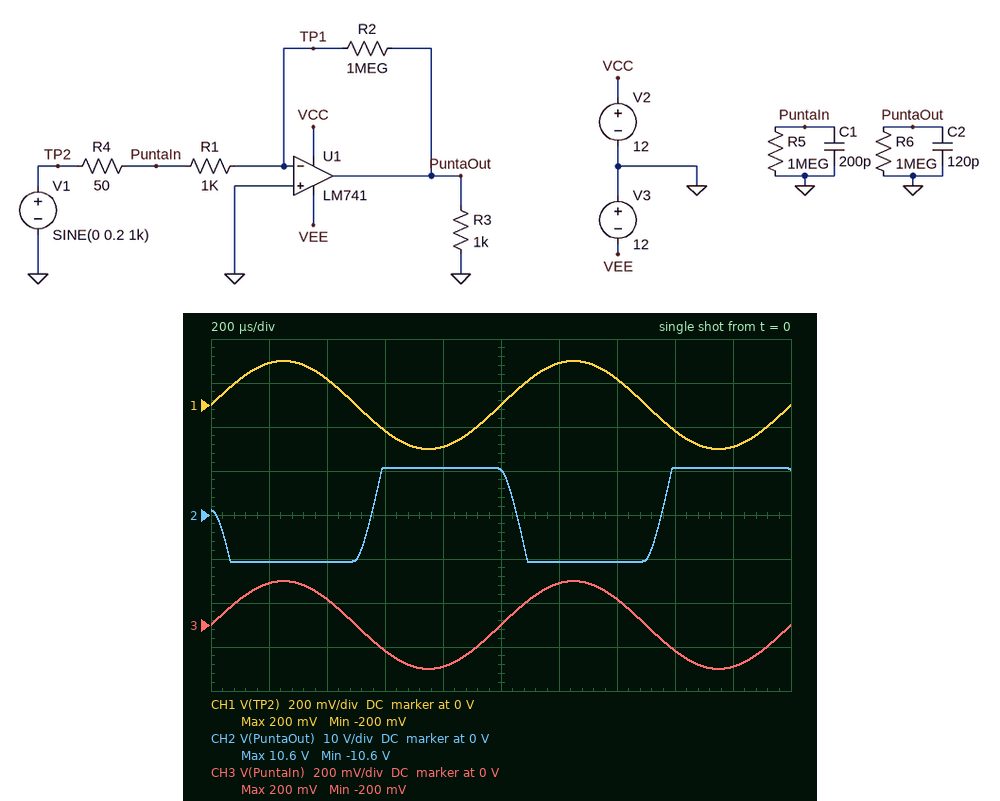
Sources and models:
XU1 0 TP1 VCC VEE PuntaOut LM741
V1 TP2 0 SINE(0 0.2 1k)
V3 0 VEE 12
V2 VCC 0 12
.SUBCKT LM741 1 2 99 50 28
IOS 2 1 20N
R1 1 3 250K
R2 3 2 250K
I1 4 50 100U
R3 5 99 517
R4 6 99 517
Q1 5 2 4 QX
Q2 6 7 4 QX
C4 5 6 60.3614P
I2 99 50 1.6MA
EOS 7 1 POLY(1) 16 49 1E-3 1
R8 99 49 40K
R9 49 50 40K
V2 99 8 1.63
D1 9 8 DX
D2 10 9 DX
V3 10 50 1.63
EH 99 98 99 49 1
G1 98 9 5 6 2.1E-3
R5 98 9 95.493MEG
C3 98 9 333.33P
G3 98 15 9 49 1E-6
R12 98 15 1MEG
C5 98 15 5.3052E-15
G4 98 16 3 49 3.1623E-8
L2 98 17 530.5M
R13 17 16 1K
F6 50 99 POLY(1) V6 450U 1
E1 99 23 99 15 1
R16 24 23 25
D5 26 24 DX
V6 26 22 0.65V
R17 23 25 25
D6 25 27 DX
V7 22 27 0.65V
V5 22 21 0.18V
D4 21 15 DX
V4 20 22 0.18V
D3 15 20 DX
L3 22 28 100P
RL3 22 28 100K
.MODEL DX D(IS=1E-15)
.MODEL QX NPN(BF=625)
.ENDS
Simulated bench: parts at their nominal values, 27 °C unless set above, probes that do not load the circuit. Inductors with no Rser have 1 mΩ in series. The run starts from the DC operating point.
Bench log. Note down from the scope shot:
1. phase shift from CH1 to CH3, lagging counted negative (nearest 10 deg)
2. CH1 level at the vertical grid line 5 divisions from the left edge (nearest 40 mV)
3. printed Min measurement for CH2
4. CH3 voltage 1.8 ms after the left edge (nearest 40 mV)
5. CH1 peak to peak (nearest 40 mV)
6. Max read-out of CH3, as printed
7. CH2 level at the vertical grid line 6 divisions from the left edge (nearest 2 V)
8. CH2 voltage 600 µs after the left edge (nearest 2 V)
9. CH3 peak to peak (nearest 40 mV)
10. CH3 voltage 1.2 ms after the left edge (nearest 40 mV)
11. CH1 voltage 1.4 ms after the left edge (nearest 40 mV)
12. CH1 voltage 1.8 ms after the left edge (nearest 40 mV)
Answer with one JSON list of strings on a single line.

["0 deg", "0 V", "-10.6 V", "-200 mV", "400 mV", "200 mV", "-10 V", "10 V", "400 mV", "200 mV", "120 mV", "-200 mV"]
